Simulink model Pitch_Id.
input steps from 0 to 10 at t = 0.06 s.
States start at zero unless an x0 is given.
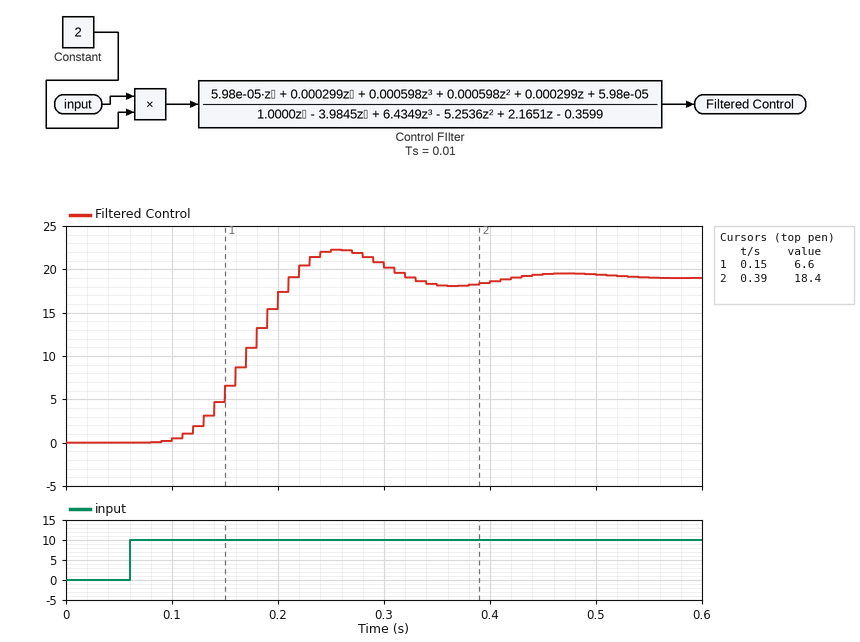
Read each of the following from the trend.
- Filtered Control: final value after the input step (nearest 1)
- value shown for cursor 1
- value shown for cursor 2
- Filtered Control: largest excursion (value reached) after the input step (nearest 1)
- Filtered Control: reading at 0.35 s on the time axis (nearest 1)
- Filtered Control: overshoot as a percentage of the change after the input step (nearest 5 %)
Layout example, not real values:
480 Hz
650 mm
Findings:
19
6.6
18.4
22
18
15 %
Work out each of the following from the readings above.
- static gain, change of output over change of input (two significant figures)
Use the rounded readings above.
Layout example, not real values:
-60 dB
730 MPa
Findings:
1.9
